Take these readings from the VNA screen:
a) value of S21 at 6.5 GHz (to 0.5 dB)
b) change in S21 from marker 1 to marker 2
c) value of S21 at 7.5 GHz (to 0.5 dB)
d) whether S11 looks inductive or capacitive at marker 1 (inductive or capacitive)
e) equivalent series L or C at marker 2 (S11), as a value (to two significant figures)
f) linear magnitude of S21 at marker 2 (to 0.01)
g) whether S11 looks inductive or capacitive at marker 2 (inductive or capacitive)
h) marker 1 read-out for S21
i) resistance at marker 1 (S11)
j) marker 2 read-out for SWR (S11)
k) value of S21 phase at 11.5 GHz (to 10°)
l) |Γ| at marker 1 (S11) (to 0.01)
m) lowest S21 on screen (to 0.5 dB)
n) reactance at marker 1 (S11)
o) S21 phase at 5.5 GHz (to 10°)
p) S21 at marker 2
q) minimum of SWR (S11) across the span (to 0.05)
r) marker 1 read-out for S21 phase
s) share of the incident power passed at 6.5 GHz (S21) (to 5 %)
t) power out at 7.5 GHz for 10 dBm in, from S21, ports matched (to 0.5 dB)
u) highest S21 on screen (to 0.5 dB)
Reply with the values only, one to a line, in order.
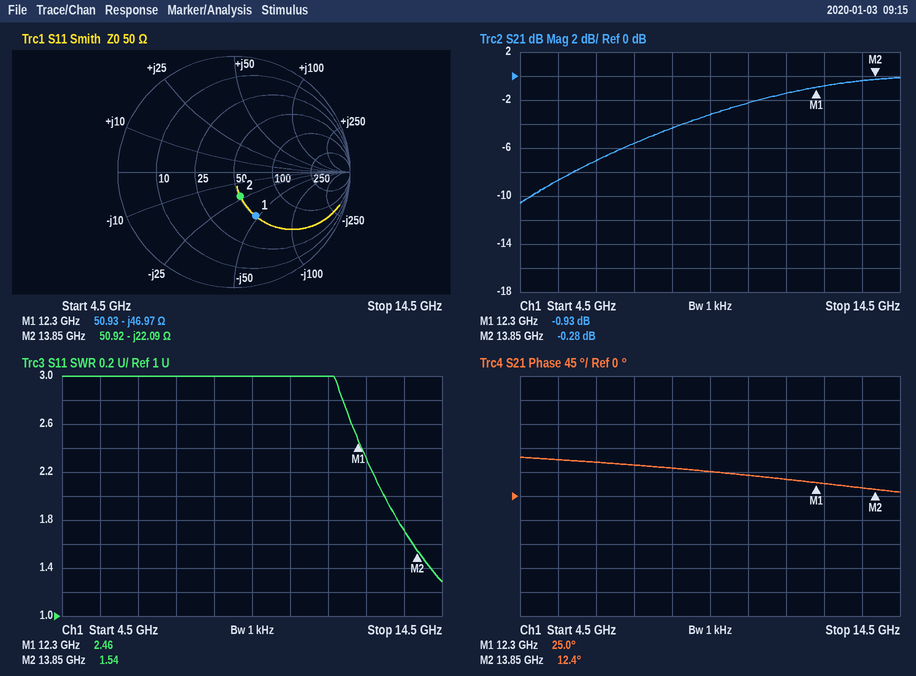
-7.0 dB
0.65 dB
-5.5 dB
capacitive
520 fF
0.97
capacitive
-0.93 dB
50.93 Ω
1.54
30°
0.42
-10.5 dB
-46.97 Ω
70°
-0.28 dB
1.30
25.0°
20 %
4.5 dBm
0.0 dB
